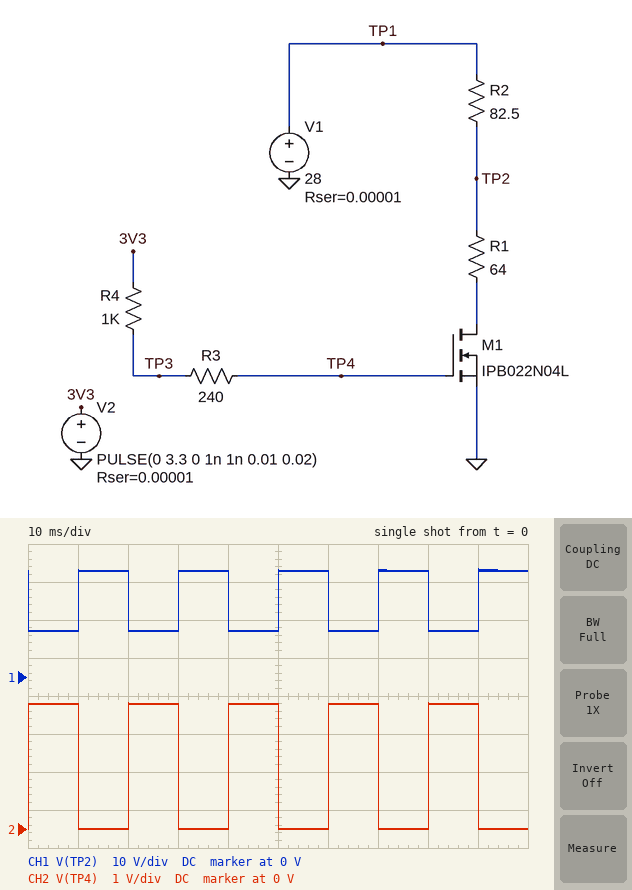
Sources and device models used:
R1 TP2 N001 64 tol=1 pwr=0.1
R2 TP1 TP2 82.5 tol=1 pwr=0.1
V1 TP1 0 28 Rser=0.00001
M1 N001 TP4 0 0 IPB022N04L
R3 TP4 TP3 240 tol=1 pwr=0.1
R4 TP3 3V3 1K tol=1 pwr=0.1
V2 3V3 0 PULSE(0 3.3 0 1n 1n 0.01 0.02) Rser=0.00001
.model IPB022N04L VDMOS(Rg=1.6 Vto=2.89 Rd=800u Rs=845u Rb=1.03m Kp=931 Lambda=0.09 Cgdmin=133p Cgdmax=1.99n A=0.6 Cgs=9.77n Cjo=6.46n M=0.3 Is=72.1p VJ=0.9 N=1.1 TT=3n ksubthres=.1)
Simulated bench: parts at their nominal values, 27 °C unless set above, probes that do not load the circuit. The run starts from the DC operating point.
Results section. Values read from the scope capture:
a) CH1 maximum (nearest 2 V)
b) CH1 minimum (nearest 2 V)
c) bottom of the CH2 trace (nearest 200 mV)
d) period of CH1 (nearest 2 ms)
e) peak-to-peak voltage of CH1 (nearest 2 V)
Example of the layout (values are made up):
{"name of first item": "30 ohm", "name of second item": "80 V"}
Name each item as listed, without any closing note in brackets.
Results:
{"CH1 maximum": "28 V", "CH1 minimum": "12 V", "bottom of the CH2 trace": "0 V", "period of CH1": "20 ms", "peak-to-peak voltage of CH1": "16 V"}
